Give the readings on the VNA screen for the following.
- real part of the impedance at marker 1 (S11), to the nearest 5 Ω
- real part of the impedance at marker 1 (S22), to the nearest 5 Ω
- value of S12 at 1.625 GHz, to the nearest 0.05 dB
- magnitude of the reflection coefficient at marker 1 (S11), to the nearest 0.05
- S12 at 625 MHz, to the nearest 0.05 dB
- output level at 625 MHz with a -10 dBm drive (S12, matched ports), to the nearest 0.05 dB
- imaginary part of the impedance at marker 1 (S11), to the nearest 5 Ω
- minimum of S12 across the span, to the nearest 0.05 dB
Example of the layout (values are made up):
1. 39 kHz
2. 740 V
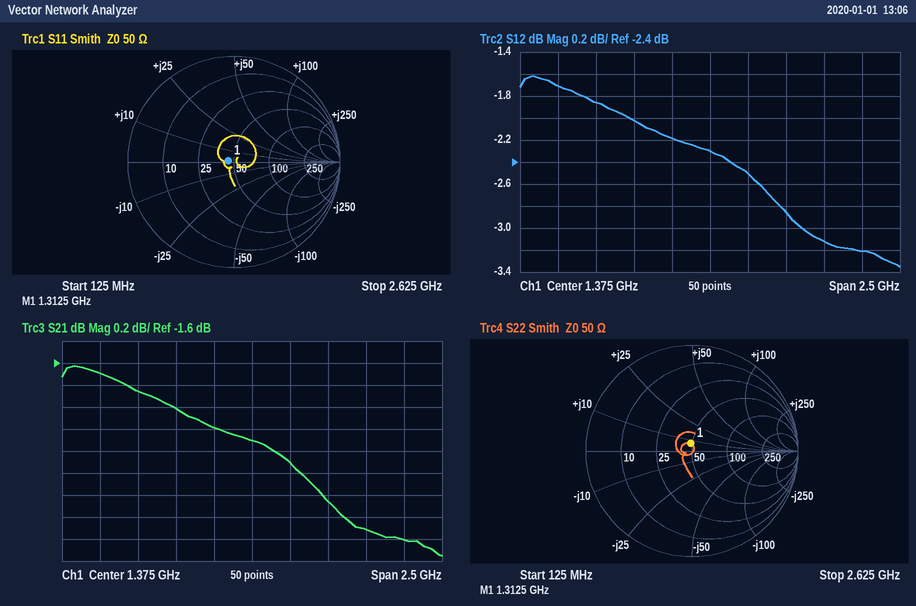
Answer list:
1. 45 Ω
2. 50 Ω
3. -2.50 dB
4. 0.05
5. -1.85 dB
6. -11.85 dBm
7. 0 Ω
8. -3.35 dB
